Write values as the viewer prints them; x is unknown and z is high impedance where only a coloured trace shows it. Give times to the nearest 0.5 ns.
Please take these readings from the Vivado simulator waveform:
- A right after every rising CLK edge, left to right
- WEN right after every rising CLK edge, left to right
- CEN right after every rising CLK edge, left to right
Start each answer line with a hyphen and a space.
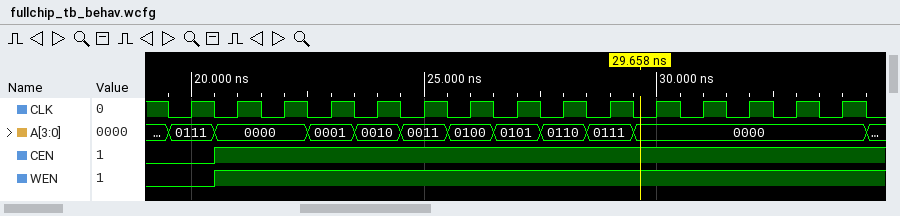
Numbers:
- 0111, 0000, 0000, 0001, 0010, 0011, 0100, 0101, 0110, 0111, 0000, 0000, 0000, 0000, 0000
- 0 1 1 1 1 1 1 1 1 1 1 1 1 1 1
- 0 1 1 1 1 1 1 1 1 1 1 1 1 1 1
